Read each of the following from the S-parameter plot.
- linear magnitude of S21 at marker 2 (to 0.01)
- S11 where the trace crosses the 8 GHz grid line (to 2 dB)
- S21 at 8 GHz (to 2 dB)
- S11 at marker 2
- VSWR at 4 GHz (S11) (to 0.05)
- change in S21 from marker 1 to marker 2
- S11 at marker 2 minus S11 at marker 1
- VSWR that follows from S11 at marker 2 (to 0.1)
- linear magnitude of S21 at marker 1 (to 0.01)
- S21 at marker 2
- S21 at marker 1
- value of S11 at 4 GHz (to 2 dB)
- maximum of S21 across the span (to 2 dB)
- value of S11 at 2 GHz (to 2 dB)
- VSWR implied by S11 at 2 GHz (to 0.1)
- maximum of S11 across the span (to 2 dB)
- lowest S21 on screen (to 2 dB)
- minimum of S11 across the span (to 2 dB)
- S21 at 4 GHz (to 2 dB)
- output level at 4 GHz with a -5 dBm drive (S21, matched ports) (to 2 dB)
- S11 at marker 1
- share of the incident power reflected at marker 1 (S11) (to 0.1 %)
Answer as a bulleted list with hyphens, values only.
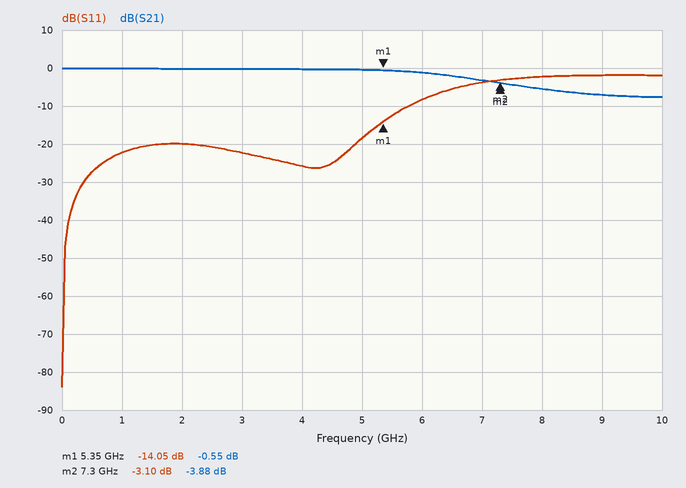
- 0.64
- -2 dB
- -6 dB
- -3.10 dB
- 1.10
- -3.33 dB
- 10.95 dB
- 5.7
- 0.94
- -3.88 dB
- -0.55 dB
- -26 dB
- 0 dB
- -20 dB
- 1.2
- -2 dB
- -8 dB
- -84 dB
- 0 dB
- -6 dBm
- -14.05 dB
- 3.9 %
